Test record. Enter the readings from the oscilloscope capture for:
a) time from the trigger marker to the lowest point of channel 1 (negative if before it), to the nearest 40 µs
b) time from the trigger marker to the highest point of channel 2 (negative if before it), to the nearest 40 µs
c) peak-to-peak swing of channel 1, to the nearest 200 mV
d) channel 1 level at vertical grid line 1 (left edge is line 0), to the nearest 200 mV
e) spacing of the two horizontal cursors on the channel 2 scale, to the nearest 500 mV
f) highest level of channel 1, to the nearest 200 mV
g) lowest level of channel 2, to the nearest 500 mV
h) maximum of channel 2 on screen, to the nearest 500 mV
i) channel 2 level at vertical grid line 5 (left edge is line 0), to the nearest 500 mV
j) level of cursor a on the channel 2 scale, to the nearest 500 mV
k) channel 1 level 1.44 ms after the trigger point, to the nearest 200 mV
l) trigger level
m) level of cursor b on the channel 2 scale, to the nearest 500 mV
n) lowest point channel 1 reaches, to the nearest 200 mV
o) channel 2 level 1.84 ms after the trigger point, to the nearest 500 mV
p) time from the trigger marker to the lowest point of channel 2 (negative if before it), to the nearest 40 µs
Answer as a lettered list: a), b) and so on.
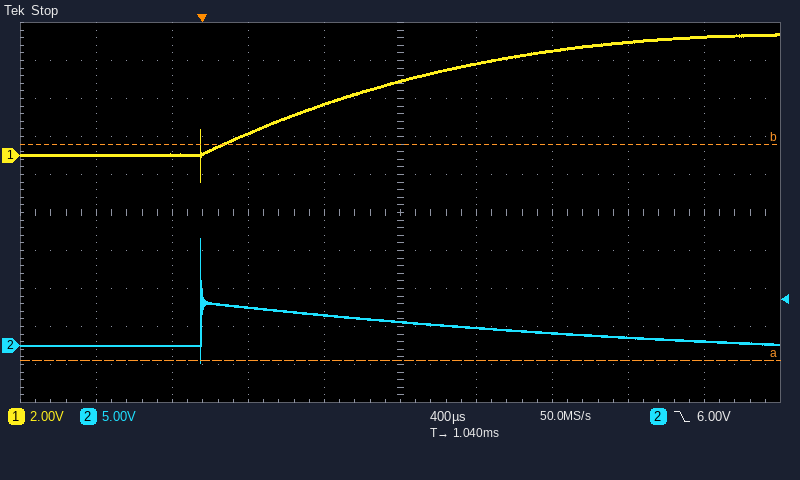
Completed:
a) 0 µs
b) 0 µs
c) 7.8 V
d) 0.0 V
e) 28.5 V
f) 6.4 V
g) -2.0 V
h) 14.0 V
i) 3.0 V
j) -2.0 V
k) 4.8 V
l) 6.00 V
m) 26.5 V
n) -1.4 V
o) 1.5 V
p) 0 µs
